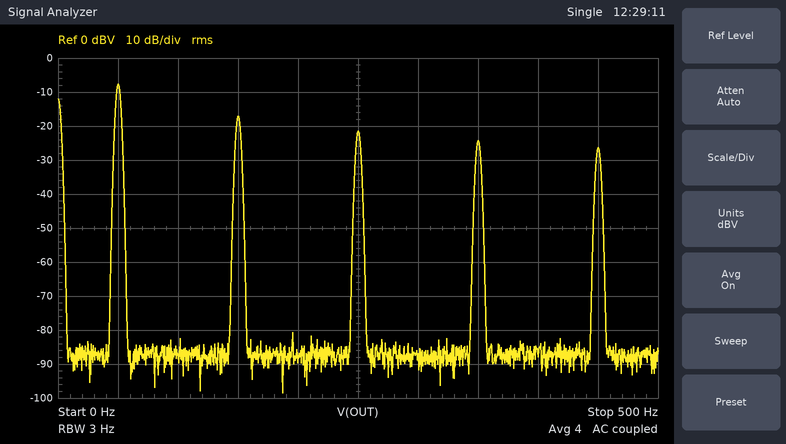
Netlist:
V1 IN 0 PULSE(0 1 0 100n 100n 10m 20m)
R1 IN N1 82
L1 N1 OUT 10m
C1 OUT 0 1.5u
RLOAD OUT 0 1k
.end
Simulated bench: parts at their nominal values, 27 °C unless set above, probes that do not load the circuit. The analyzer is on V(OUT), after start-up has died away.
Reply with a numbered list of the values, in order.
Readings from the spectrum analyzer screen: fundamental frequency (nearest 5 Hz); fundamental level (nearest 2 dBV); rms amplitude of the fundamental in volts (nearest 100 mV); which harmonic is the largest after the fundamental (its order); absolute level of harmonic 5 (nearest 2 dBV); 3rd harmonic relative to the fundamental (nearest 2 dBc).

1. 50 Hz
2. -8 dBV
3. 400 mV
4. 3
5. -22 dBV
6. -10 dBc
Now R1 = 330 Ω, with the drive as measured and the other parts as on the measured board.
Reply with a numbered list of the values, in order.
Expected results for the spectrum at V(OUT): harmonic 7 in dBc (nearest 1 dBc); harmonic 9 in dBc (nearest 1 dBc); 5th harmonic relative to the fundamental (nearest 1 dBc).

1. -19 dBc
2. -22 dBc
3. -15 dBc
